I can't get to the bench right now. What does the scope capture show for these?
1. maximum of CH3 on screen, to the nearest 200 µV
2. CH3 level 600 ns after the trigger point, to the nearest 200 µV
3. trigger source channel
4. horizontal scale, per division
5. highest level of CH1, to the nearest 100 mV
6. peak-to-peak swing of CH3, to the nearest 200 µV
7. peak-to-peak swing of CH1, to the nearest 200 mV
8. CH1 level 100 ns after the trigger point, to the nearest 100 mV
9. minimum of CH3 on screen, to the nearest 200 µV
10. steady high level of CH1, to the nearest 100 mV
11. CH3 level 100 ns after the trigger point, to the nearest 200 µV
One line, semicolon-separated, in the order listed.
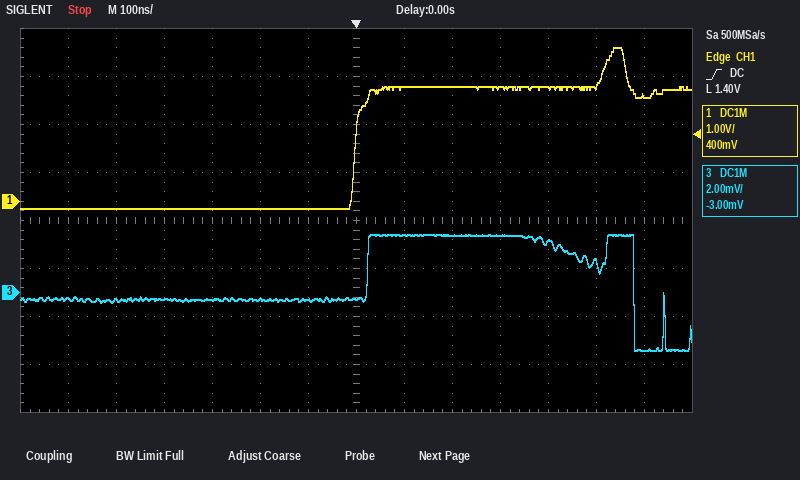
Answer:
2.4 mV; -2.4 mV; CH1; 100 ns; 3.2 V; 4.8 mV; 3.4 V; 2.4 V; -2.4 mV; 2.4 V; 2.4 mV
